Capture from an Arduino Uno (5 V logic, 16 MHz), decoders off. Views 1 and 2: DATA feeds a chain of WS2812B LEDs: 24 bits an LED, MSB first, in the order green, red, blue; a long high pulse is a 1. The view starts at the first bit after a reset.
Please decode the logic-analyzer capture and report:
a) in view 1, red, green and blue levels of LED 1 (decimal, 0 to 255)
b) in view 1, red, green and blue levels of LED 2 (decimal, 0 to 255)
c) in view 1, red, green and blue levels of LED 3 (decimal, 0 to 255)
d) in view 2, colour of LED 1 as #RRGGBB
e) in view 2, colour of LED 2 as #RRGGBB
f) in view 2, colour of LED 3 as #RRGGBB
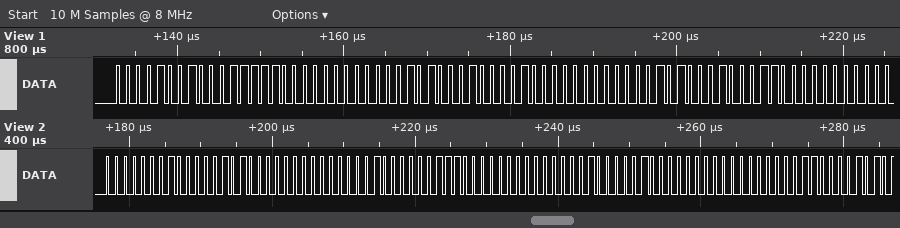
31, 9, 0
33, 10, 0
35, 10, 0
#050100
#070200
#080200
